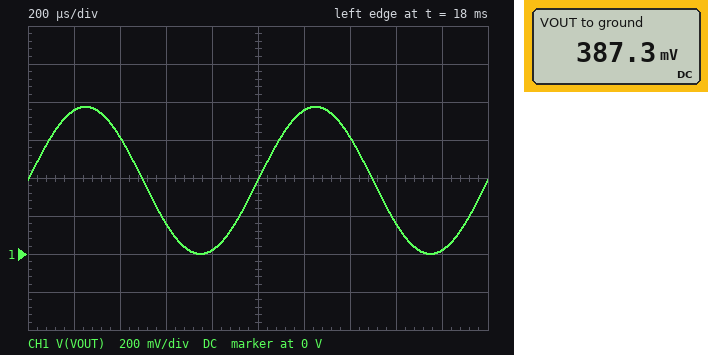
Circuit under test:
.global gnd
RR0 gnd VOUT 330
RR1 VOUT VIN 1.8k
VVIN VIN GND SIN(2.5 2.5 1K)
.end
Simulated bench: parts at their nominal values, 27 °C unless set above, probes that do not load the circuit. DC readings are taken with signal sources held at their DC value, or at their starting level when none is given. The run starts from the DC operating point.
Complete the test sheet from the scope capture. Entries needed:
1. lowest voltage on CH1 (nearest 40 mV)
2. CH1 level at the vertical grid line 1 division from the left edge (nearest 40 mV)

0 V
760 mV
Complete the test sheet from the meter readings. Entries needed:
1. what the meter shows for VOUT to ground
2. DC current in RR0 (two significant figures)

387.3 mV
1.2 mA
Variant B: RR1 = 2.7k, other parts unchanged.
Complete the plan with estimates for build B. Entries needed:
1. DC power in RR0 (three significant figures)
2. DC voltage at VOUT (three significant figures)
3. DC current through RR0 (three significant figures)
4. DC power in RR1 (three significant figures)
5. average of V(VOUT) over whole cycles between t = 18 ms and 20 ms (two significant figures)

225 µW
272 mV
825 µA
1.84 mW
270 mV
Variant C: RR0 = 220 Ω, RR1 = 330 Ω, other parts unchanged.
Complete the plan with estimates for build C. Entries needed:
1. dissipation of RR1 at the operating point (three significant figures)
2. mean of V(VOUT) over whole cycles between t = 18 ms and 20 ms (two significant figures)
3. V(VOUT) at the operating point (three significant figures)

6.82 mW
1.0 V
1.00 V
